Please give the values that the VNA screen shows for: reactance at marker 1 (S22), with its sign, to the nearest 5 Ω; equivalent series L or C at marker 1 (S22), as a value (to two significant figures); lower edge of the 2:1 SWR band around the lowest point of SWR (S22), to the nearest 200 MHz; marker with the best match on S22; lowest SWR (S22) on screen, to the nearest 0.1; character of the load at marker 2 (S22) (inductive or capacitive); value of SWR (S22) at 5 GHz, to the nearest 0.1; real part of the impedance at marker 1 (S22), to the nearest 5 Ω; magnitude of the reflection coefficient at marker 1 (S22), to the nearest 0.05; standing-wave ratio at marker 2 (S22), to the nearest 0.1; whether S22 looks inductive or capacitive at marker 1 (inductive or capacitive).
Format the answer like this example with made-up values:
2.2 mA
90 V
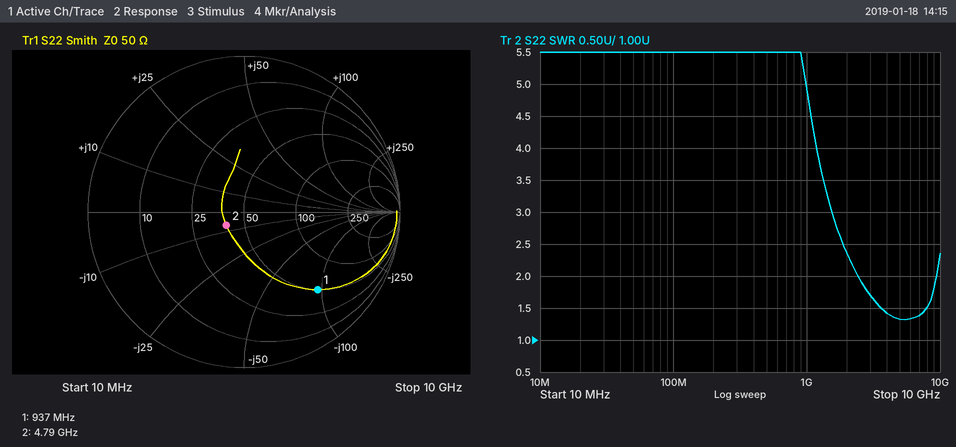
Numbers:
-95 Ω
1.8 pF
2.4 GHz
marker 2
1.3
capacitive
1.3
50 Ω
0.70
1.3
capacitive
